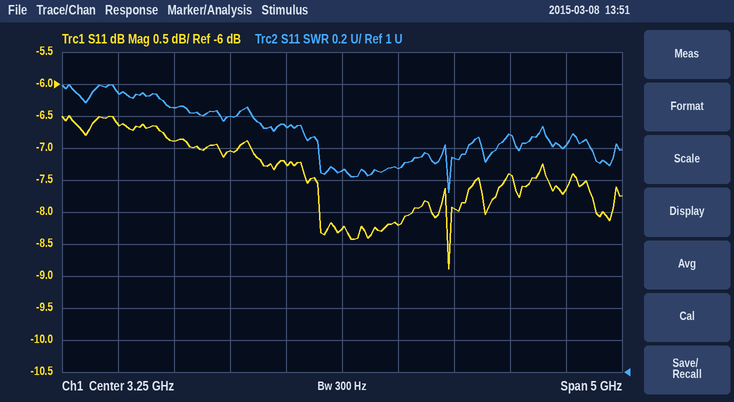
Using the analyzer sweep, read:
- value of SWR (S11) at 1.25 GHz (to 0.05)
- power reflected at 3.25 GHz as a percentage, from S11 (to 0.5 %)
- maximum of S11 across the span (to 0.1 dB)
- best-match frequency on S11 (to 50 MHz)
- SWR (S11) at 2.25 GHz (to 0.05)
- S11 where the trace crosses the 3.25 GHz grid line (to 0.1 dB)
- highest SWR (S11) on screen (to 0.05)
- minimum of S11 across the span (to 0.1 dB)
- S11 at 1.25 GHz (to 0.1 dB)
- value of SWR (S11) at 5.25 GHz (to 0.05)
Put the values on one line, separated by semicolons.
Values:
2.75; 15.0 %; -6.5 dB; 4.20 GHz; 2.60; -8.3 dB; 2.80; -8.9 dB; -6.6 dB; 2.40
